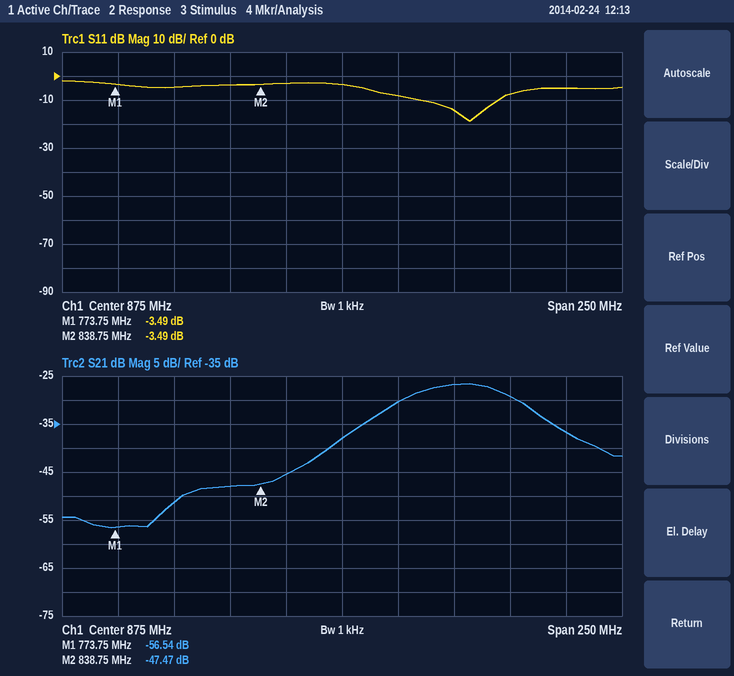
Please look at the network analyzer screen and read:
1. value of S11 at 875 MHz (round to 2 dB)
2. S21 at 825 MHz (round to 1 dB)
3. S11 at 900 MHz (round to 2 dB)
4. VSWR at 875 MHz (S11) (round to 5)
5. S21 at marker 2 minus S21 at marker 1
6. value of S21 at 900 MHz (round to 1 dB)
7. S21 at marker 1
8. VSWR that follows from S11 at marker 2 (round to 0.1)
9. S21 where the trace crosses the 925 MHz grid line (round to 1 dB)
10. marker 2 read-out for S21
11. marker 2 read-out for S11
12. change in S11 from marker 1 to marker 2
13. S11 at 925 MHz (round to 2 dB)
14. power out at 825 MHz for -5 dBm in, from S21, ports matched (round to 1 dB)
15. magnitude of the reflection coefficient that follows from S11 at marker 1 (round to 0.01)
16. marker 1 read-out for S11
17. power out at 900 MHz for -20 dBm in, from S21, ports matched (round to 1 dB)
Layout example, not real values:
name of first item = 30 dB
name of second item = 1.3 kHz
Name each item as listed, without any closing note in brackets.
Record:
value of S11 at 875 MHz = -4 dB
S21 at 825 MHz = -48 dB
S11 at 900 MHz = -8 dB
VSWR at 875 MHz (S11) = 5
S21 at marker 2 minus S21 at marker 1 = 9.07 dB
value of S21 at 900 MHz = -30 dB
S21 at marker 1 = -56.54 dB
VSWR that follows from S11 at marker 2 = 5.0
S21 where the trace crosses the 925 MHz grid line = -27 dB
marker 2 read-out for S21 = -47.47 dB
marker 2 read-out for S11 = -3.49 dB
change in S11 from marker 1 to marker 2 = 0.00 dB
S11 at 925 MHz = -14 dB
power out at 825 MHz for -5 dBm in, from S21, ports matched = -53 dBm
magnitude of the reflection coefficient that follows from S11 at marker 1 = 0.67
marker 1 read-out for S11 = -3.49 dB
power out at 900 MHz for -20 dBm in, from S21, ports matched = -50 dBm
